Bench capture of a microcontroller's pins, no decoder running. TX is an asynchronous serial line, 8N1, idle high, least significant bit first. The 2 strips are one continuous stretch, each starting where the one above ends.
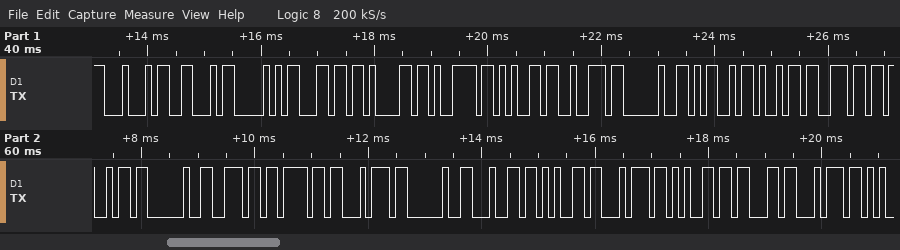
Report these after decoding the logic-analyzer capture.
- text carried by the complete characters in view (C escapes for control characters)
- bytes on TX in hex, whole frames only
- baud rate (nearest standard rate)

"DFPlayer Mini not detect"
44 46 50 6C 61 79 65 72 20 4D 69 6E 69 20 6E 6F 74 20 64 65 74 65 63 74
9600 baud
